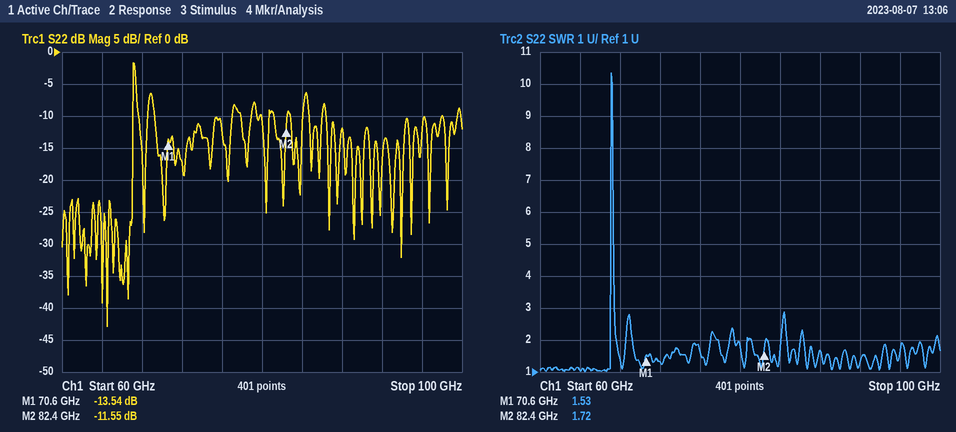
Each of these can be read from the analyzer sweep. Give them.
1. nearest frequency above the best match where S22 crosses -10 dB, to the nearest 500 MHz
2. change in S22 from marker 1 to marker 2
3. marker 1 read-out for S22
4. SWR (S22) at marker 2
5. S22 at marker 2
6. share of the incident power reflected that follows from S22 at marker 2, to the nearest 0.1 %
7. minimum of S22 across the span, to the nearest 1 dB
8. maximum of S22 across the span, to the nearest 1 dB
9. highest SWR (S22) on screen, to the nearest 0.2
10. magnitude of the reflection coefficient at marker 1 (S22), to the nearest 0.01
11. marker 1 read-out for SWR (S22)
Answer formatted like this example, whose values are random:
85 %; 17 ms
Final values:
67.0 GHz; 1.99 dB; -13.54 dB; 1.72; -11.55 dB; 7.0 %; -43 dB; -2 dB; 10.4; 0.21; 1.53
